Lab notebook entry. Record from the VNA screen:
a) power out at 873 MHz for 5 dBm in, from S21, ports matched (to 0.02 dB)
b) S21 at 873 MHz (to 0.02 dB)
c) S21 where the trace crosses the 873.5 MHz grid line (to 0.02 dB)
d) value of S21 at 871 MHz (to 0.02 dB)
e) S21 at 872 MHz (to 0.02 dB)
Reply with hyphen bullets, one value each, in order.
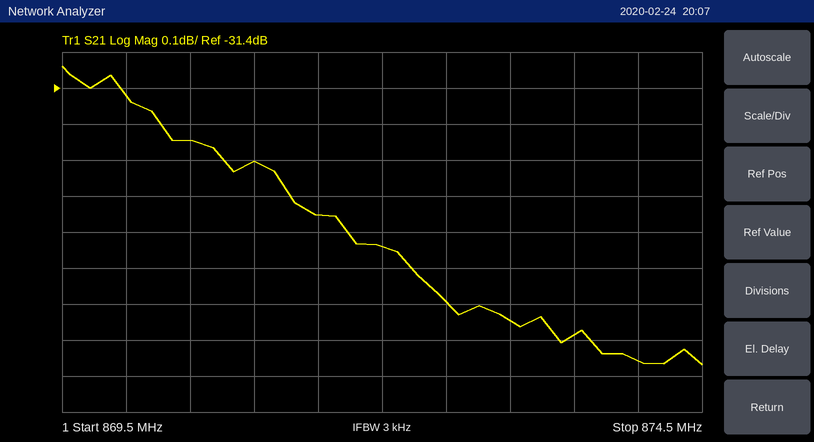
- -27.04 dBm
- -32.04 dB
- -32.08 dB
- -31.60 dB
- -31.84 dB
